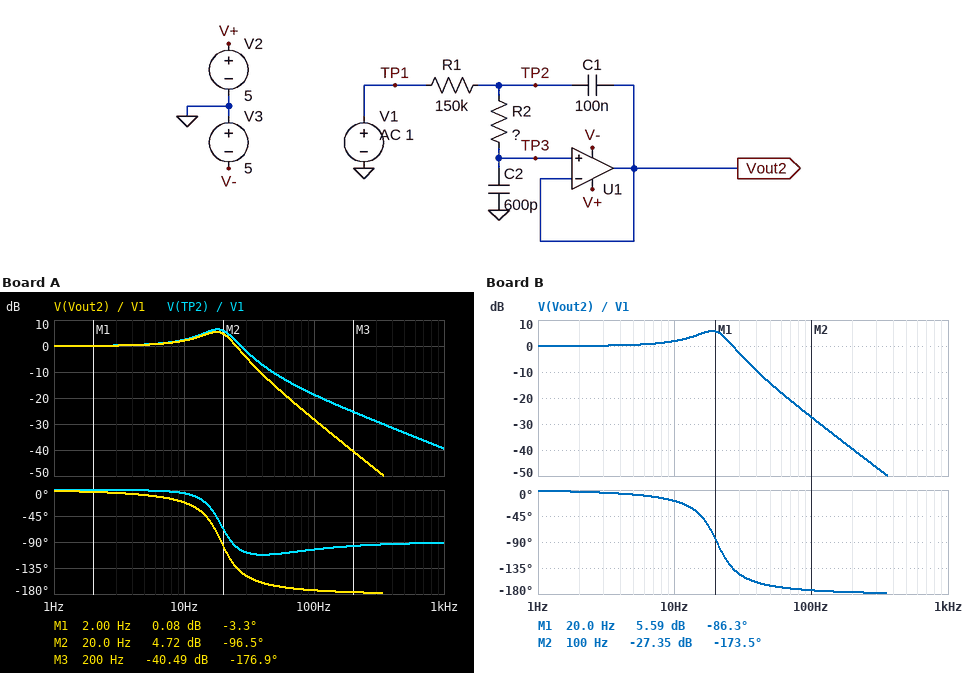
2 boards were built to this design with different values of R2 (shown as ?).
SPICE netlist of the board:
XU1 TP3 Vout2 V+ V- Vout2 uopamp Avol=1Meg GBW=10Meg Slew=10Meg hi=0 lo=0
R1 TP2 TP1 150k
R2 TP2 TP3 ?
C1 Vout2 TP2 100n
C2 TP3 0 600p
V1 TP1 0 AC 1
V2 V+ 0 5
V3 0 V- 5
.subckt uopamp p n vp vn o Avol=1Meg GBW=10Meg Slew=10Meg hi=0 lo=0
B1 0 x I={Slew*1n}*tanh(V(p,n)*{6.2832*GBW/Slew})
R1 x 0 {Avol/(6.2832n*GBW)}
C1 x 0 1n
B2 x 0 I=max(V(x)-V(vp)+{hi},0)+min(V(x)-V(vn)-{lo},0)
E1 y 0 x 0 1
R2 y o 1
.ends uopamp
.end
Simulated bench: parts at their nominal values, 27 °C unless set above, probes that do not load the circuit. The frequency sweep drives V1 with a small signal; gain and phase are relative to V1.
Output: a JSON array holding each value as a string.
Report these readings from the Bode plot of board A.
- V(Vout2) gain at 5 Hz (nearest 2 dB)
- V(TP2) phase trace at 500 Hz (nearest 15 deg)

["0 dB", "-90 deg"]
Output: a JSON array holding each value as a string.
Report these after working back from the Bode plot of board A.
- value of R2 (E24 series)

["7.5 MΩ"]
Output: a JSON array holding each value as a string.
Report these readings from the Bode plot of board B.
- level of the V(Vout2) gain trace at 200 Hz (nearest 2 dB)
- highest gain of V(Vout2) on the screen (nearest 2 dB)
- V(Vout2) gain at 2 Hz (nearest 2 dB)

["-40 dB", "6 dB", "0 dB"]
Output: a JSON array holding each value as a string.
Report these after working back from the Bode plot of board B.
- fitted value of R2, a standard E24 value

["6.8 MΩ"]
